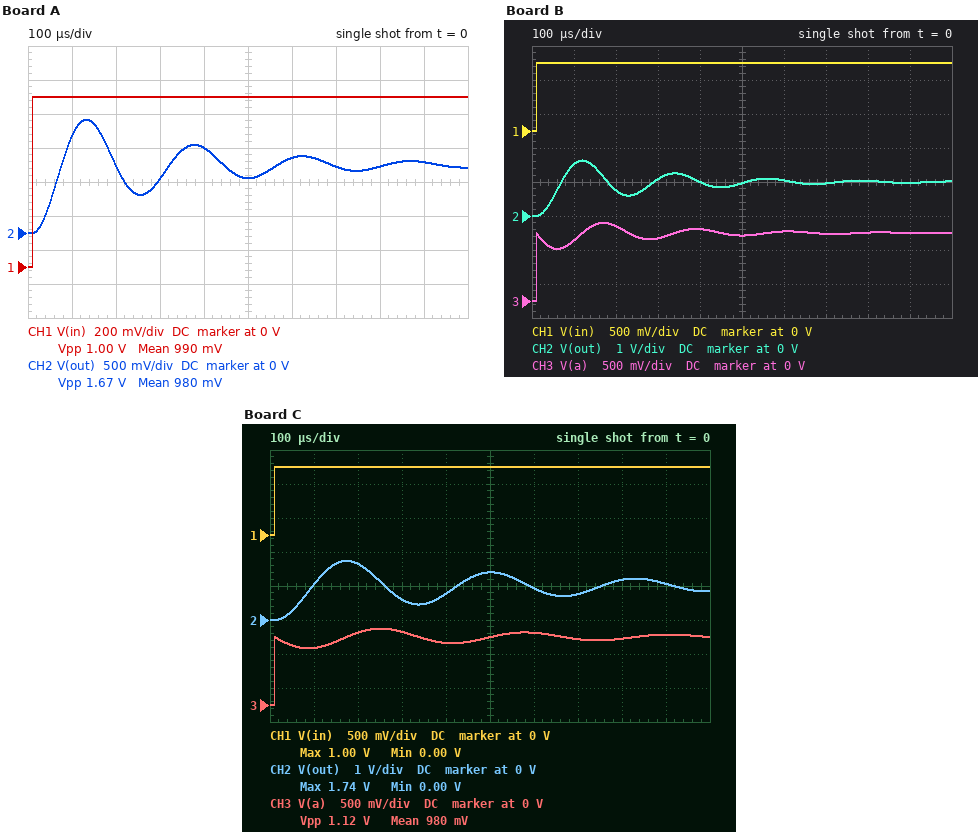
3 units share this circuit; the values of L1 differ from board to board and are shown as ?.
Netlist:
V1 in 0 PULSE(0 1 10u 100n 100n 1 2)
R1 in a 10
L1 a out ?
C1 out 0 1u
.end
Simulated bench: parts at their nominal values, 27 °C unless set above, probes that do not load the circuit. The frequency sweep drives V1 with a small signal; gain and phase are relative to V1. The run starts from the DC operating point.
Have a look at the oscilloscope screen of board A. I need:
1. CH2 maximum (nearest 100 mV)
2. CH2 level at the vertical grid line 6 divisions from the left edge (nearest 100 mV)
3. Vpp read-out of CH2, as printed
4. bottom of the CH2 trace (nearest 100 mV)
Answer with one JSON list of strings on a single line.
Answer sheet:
["1.7 V", "1.1 V", "1.67 V", "0 V"]
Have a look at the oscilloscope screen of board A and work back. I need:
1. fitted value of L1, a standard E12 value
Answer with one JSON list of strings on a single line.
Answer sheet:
["1.5 mH"]
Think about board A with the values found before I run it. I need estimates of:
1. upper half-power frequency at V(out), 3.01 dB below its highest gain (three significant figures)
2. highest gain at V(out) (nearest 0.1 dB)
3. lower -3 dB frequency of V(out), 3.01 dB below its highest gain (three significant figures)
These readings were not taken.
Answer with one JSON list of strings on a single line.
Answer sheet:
["4.54 kHz", "11.8 dB", "3.46 kHz"]
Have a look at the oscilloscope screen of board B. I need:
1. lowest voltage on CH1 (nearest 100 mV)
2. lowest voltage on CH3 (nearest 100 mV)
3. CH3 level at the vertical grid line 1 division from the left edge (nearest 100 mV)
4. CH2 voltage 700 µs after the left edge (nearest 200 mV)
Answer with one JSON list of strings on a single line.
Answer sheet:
["0 V", "0 V", "900 mV", "1.0 V"]
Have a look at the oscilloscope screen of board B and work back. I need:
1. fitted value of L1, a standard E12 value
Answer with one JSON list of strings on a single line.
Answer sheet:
["1.2 mH"]
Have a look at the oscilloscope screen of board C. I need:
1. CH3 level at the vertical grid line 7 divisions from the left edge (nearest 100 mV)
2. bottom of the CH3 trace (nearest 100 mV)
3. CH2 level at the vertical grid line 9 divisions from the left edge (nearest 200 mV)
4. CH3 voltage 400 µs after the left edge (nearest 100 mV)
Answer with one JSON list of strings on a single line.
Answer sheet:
["1.0 V", "0 V", "1.0 V", "900 mV"]
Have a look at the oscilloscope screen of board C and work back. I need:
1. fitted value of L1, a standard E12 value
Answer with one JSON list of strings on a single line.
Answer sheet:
["2.7 mH"]
